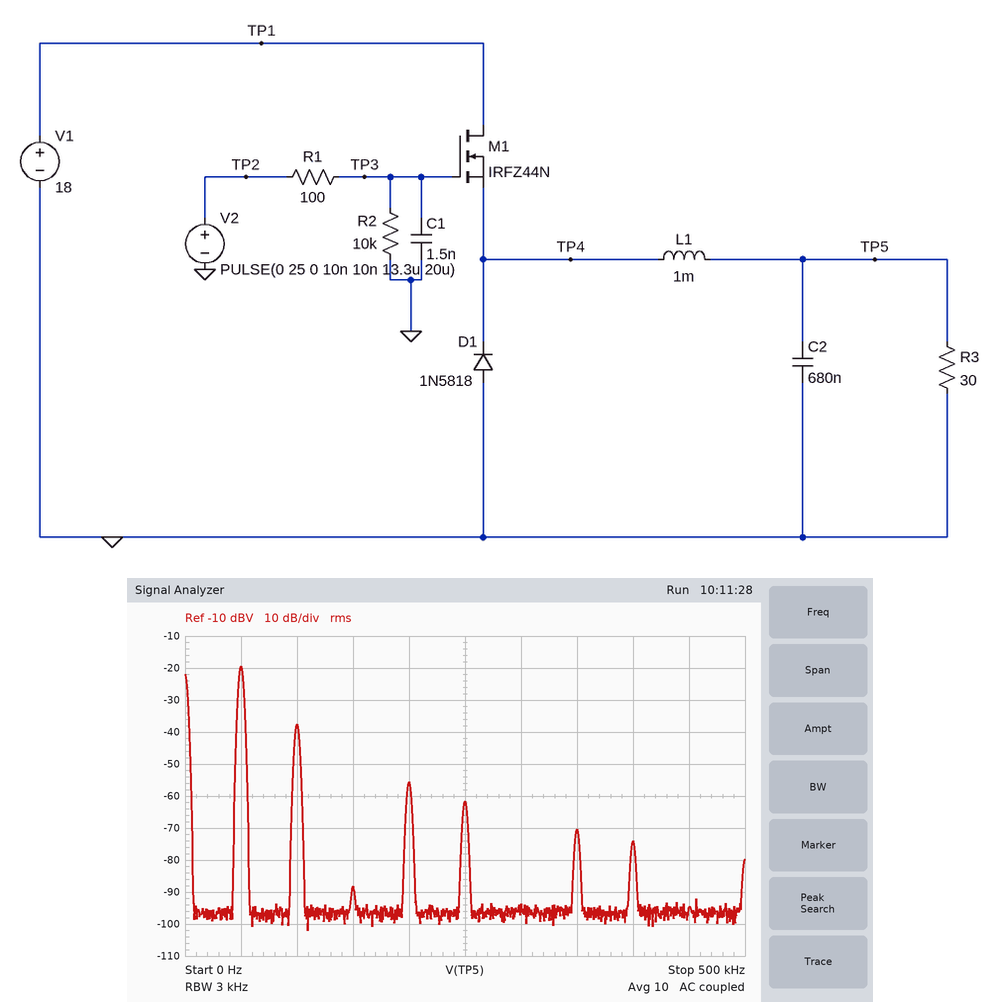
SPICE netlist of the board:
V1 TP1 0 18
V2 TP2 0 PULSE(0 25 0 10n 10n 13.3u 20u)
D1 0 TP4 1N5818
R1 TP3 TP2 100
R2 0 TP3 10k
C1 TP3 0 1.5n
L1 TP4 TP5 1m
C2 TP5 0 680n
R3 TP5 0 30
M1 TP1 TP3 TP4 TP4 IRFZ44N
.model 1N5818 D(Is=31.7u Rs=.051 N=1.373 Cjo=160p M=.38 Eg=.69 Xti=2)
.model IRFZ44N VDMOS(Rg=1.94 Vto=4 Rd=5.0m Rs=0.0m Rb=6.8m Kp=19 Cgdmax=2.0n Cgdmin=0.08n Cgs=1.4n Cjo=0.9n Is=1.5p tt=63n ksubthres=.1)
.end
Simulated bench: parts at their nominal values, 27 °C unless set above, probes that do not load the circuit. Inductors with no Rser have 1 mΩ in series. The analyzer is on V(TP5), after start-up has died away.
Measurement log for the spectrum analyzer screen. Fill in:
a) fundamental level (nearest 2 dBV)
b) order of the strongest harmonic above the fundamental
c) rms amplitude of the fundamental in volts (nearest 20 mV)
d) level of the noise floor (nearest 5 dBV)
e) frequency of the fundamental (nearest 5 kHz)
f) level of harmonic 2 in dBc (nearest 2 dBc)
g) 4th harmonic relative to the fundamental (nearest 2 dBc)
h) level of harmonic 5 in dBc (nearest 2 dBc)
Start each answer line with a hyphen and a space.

- -20 dBV
- 2
- 100 mV
- -95 dBV
- 50 kHz
- -18 dBc
- -36 dBc
- -42 dBc
